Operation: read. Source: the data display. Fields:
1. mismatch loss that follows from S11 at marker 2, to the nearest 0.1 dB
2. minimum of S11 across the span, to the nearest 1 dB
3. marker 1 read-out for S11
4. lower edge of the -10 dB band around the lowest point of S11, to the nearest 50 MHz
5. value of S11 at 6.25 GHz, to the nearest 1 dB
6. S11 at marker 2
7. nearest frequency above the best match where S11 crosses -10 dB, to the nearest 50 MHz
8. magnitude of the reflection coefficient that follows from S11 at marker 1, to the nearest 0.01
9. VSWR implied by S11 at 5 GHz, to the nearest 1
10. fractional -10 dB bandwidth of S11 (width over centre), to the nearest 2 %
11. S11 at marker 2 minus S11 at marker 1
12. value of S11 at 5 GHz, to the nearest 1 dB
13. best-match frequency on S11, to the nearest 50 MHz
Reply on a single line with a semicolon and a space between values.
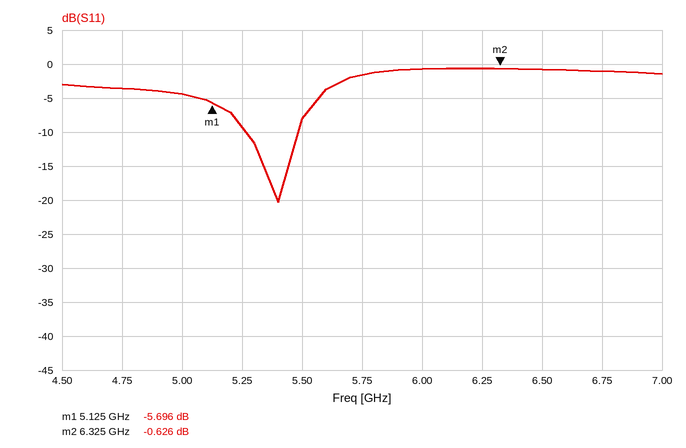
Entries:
8.7 dB; -20 dB; -5.696 dB; 5.25 GHz; -1 dB; -0.626 dB; 5.50 GHz; 0.52; 4; 4 %; 5.070 dB; -4 dB; 5.40 GHz
